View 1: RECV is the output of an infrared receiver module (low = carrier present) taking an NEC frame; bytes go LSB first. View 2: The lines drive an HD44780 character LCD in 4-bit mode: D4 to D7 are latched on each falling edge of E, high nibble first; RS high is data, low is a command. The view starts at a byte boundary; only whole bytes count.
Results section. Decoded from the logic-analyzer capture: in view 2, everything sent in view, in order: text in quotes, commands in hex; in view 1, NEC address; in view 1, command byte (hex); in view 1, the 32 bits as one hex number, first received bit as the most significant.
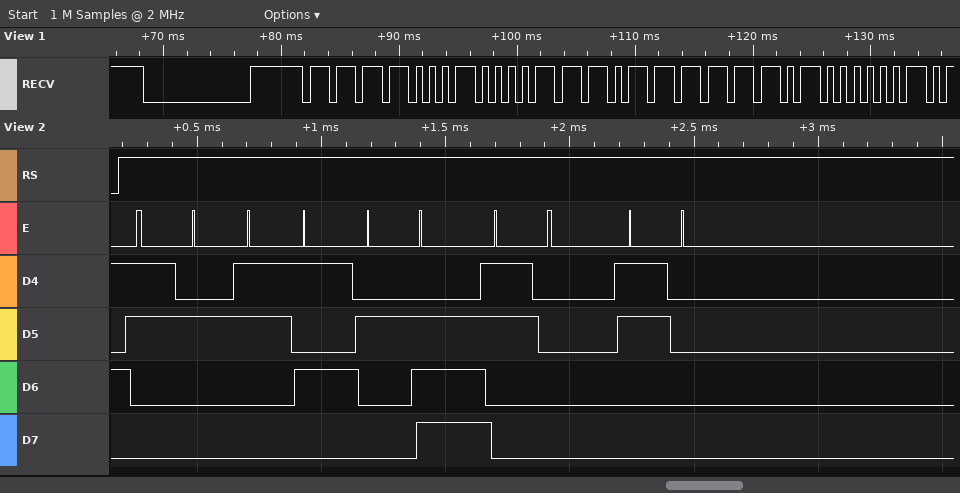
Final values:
"25.00"
0x8F
0xBF
0xF10EFD02
